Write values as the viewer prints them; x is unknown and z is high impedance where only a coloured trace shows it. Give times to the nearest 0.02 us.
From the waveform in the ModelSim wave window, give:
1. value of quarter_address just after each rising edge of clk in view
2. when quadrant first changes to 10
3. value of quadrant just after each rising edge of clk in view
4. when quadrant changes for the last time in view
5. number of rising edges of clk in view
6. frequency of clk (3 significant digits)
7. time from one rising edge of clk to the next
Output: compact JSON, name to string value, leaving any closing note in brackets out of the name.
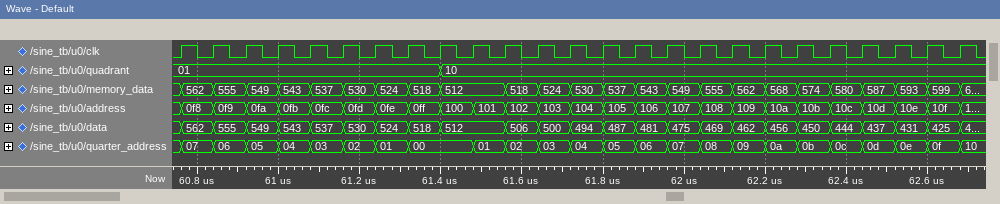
{"value of quarter_address just after each rising edge of clk in view": "07, 06, 05, 04, 03, 02, 01, 00, 00, 01, 02, 03, 04, 05, 06, 07, 08, 09, 0a, 0b, 0c, 0d, 0e, 0f, 10", "when quadrant first changes to 10": "61.4 us", "value of quadrant just after each rising edge of clk in view": "01, 01, 01, 01, 01, 01, 01, 01, 10, 10, 10, 10, 10, 10, 10, 10, 10, 10, 10, 10, 10, 10, 10, 10, 10", "when quadrant changes for the last time in view": "61.4 us", "number of rising edges of clk in view": "25", "frequency of clk": "12.5 MHz", "time from one rising edge of clk to the next": "0.08 us"}
